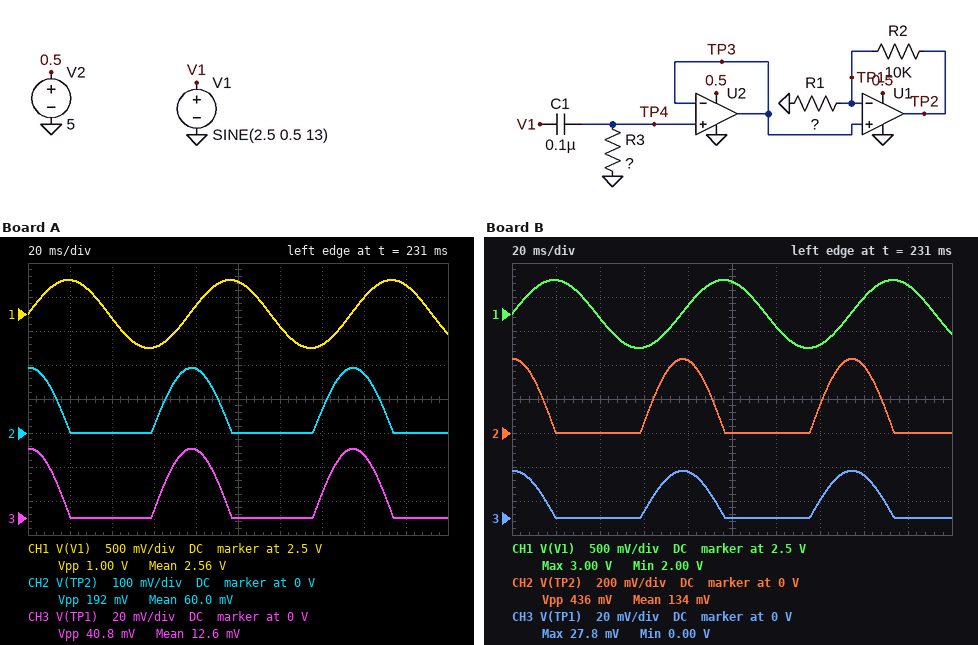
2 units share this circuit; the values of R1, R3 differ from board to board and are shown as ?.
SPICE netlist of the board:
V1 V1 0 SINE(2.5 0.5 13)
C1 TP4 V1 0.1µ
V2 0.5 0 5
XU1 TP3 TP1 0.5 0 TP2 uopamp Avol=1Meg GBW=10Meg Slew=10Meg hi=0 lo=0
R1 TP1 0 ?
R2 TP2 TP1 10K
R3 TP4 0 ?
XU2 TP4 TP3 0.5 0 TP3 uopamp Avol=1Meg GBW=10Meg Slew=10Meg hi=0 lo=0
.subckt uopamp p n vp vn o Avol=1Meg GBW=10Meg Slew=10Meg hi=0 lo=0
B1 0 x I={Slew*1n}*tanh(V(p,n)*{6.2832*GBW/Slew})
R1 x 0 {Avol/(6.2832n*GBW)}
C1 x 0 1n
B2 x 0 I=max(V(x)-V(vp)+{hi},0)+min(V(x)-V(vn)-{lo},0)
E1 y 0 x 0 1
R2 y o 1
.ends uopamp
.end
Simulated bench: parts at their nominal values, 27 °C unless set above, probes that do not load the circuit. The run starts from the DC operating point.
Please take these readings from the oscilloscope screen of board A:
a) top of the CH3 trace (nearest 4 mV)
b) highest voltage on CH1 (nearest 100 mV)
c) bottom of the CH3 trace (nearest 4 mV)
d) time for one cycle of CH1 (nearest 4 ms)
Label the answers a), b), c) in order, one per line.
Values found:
a) 40 mV
b) 3.0 V
c) 0 V
d) 76 ms
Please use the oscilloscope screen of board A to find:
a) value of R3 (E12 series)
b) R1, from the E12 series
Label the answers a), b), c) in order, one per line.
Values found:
a) 10 kΩ
b) 2.7 kΩ
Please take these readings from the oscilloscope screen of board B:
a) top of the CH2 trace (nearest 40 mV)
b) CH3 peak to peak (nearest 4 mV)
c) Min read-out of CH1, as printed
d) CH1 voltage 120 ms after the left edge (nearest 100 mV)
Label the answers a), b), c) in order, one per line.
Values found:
a) 440 mV
b) 28 mV
c) 2.00 V
d) 2.3 V
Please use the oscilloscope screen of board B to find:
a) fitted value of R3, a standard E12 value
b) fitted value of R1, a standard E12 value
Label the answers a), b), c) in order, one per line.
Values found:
a) 6.8 kΩ
b) 680 Ω
